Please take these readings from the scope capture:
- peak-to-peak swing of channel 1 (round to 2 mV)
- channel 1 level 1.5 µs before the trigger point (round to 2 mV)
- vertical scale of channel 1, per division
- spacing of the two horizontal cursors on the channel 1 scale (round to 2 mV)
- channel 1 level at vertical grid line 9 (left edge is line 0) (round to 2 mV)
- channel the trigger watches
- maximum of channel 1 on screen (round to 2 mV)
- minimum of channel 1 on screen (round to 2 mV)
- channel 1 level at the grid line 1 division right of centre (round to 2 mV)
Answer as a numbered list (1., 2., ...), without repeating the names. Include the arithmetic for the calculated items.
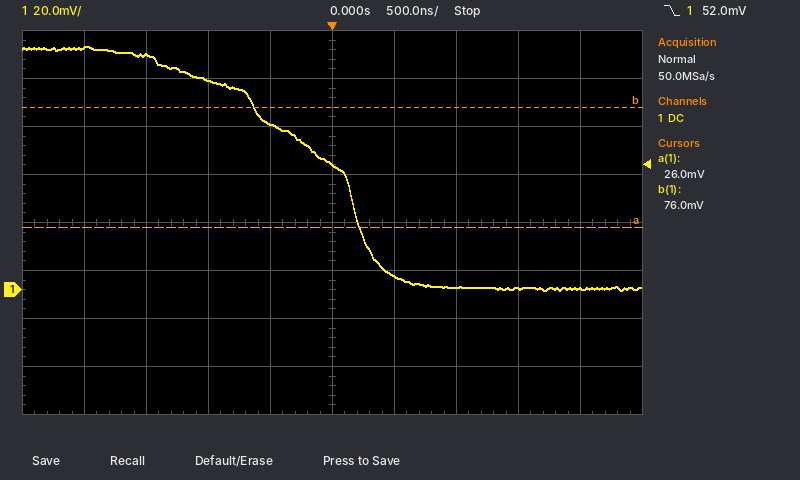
1. 102 mV − (0 mV) = 102 mV
2. 98 mV
3. 20 mV
4. 50 mV
5. 0 mV
6. channel 1
7. 102 mV
8. 0 mV
9. 6 mV
